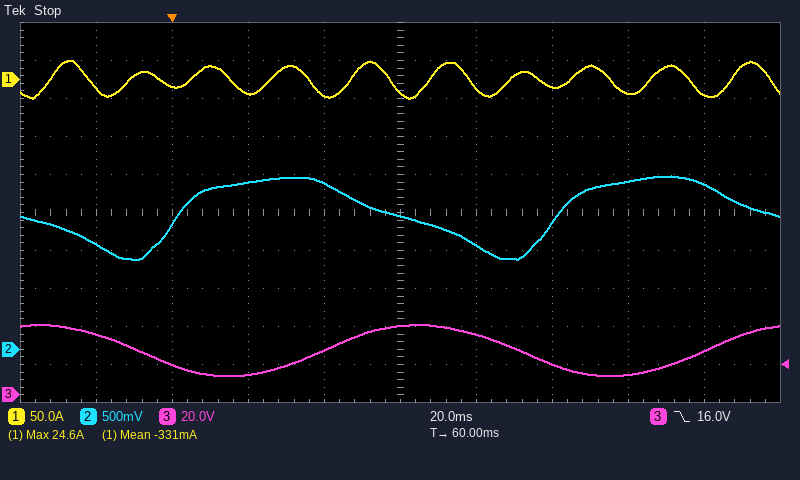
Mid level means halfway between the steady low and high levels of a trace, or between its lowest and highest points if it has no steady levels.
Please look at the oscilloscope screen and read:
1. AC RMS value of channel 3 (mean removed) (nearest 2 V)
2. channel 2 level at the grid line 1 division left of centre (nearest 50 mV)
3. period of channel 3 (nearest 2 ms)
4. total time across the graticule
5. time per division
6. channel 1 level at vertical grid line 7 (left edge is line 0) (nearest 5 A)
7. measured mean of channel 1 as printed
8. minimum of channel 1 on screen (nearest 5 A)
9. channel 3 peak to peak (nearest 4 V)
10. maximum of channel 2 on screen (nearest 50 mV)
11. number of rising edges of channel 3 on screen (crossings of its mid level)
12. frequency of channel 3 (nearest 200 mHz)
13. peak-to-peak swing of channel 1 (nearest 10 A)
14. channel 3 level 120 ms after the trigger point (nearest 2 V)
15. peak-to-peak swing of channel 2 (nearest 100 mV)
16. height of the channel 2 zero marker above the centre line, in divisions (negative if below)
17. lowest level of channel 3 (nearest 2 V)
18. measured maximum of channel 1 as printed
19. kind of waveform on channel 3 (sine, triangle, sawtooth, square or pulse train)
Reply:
10 V
2.20 V
100 ms
200 ms
20 ms
-10 A
-331 mA
-25 A
28 V
2.30 V
2
10.0 Hz
50 A
10 V
1.10 V
-3.6 div
10 V
24.6 A
sine
